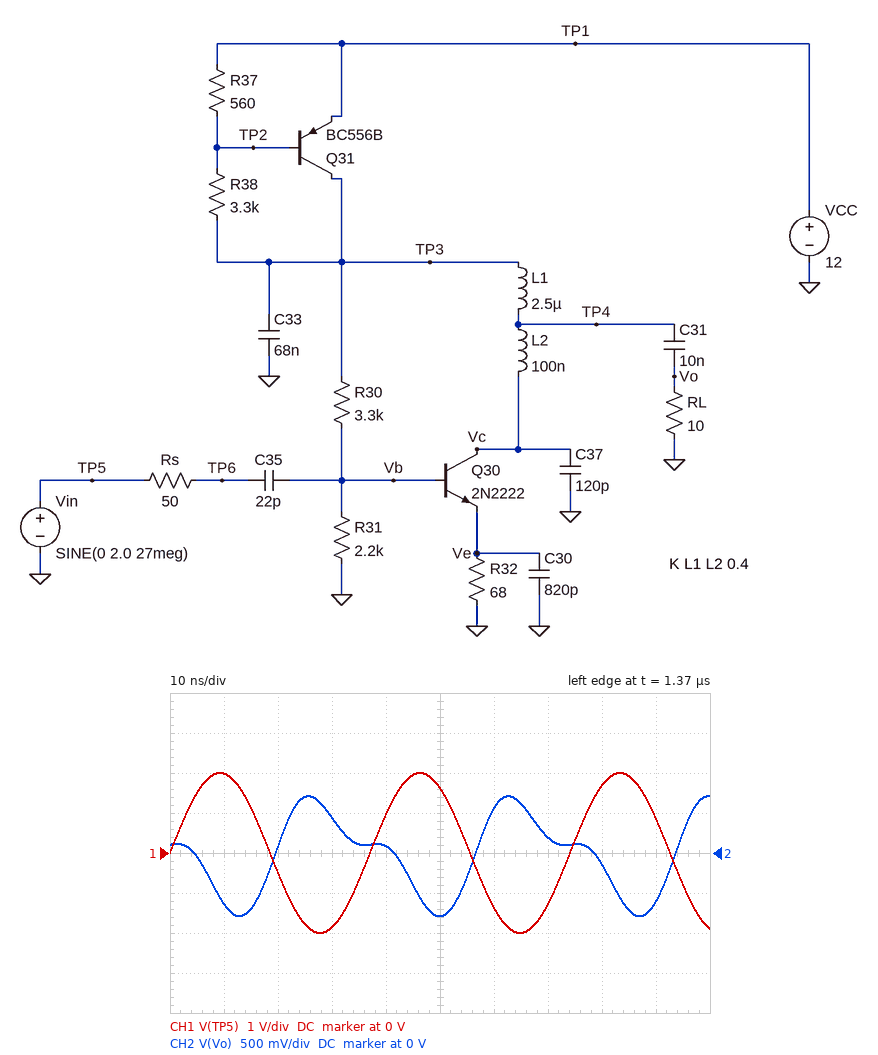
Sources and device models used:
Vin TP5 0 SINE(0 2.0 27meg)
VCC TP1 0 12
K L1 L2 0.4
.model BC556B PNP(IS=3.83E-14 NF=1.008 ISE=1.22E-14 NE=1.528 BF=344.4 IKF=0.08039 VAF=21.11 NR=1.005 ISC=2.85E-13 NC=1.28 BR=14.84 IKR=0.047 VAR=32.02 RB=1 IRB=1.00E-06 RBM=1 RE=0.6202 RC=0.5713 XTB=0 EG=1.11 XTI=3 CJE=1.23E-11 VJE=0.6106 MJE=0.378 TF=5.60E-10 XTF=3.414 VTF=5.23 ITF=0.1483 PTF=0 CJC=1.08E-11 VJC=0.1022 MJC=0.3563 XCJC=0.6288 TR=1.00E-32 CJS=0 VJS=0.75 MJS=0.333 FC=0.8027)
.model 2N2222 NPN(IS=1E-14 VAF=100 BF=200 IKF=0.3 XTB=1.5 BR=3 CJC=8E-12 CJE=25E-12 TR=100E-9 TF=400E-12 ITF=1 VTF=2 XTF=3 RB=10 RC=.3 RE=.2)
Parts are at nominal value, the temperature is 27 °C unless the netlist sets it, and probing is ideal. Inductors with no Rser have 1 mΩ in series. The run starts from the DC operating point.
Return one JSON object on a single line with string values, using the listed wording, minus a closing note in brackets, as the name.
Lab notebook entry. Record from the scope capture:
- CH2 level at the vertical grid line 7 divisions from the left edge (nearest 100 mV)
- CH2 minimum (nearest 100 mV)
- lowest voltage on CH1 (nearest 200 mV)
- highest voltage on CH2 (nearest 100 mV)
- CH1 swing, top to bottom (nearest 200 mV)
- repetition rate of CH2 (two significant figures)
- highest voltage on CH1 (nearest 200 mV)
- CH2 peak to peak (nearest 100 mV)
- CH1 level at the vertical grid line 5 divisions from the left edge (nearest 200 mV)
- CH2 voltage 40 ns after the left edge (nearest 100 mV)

{"CH2 level at the vertical grid line 7 divisions from the left edge": "200 mV", "CH2 minimum": "-800 mV", "lowest voltage on CH1": "-2.0 V", "highest voltage on CH2": "700 mV", "CH1 swing, top to bottom": "4.0 V", "repetition rate of CH2": "27 MHz", "highest voltage on CH1": "2.0 V", "CH2 peak to peak": "1.5 V", "CH1 level at the vertical grid line 5 divisions from the left edge": "1.6 V", "CH2 voltage 40 ns after the left edge": "100 mV"}
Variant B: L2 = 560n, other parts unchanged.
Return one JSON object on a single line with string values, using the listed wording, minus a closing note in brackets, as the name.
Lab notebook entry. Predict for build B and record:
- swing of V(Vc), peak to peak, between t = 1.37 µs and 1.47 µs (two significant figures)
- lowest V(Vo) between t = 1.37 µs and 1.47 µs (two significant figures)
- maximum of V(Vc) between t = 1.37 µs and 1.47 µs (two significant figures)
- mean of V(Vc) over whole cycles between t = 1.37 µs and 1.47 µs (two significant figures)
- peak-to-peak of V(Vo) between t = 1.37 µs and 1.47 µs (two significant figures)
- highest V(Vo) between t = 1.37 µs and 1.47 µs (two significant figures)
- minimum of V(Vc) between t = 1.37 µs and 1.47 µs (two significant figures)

{"swing of V(Vc), peak to peak, between t = 1.37 µs and 1.47 µs": "8.3 V", "lowest V(Vo) between t = 1.37 µs and 1.47 µs": "-590 mV", "maximum of V(Vc) between t = 1.37 µs and 1.47 µs": "11 V", "mean of V(Vc) over whole cycles between t = 1.37 µs and 1.47 µs": "6.7 V", "peak-to-peak of V(Vo) between t = 1.37 µs and 1.47 µs": "1.2 V", "highest V(Vo) between t = 1.37 µs and 1.47 µs": "630 mV", "minimum of V(Vc) between t = 1.37 µs and 1.47 µs": "2.5 V"}
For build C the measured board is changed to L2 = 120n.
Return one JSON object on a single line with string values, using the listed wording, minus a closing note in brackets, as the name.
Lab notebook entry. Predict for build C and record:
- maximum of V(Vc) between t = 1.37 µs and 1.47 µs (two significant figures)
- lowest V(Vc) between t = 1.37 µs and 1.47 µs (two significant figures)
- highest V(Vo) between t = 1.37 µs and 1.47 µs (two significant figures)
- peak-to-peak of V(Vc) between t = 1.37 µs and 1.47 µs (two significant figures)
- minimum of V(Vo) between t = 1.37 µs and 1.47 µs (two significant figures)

{"maximum of V(Vc) between t = 1.37 µs and 1.47 µs": "8.6 V", "lowest V(Vc) between t = 1.37 µs and 1.47 µs": "5.2 V", "highest V(Vo) between t = 1.37 µs and 1.47 µs": "760 mV", "peak-to-peak of V(Vc) between t = 1.37 µs and 1.47 µs": "3.4 V", "minimum of V(Vo) between t = 1.37 µs and 1.47 µs": "-770 mV"}
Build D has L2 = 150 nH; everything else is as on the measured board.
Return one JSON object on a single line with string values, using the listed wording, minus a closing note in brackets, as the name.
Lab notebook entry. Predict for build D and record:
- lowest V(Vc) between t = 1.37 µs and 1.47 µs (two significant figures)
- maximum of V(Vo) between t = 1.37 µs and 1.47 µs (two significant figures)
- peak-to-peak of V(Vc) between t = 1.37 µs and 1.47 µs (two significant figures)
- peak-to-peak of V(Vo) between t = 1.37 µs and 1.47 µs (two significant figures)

{"lowest V(Vc) between t = 1.37 µs and 1.47 µs": "5.1 V", "maximum of V(Vo) between t = 1.37 µs and 1.47 µs": "820 mV", "peak-to-peak of V(Vc) between t = 1.37 µs and 1.47 µs": "3.9 V", "peak-to-peak of V(Vo) between t = 1.37 µs and 1.47 µs": "1.6 V"}
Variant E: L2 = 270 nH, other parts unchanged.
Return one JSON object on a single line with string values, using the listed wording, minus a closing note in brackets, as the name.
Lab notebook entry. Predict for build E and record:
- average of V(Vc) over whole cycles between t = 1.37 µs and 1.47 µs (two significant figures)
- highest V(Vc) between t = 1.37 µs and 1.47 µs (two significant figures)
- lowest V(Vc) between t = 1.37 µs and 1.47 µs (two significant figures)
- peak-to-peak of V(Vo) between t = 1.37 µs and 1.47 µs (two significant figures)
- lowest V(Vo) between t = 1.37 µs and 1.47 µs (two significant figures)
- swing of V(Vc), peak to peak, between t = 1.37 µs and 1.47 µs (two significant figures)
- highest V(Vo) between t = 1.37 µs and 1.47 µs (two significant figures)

{"average of V(Vc) over whole cycles between t = 1.37 µs and 1.47 µs": "6.7 V", "highest V(Vc) between t = 1.37 µs and 1.47 µs": "11 V", "lowest V(Vc) between t = 1.37 µs and 1.47 µs": "2.5 V", "peak-to-peak of V(Vo) between t = 1.37 µs and 1.47 µs": "2.4 V", "lowest V(Vo) between t = 1.37 µs and 1.47 µs": "-1.2 V", "swing of V(Vc), peak to peak, between t = 1.37 µs and 1.47 µs": "8.6 V", "highest V(Vo) between t = 1.37 µs and 1.47 µs": "1.2 V"}
